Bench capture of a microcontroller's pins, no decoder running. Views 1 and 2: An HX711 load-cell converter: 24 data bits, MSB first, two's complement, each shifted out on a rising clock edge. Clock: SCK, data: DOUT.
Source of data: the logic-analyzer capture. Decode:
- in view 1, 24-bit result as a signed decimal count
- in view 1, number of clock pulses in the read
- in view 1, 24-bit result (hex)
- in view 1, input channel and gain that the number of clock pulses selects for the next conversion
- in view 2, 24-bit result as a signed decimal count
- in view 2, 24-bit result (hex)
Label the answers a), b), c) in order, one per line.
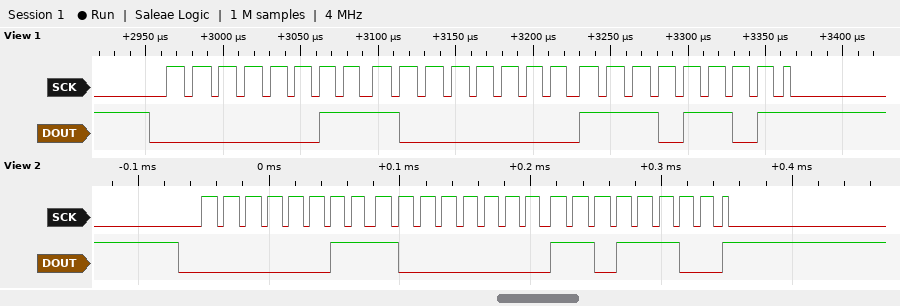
a) 229613
b) 25
c) 0x0380ED
d) channel A, gain 128
e) 229596
f) 0x0380DC
